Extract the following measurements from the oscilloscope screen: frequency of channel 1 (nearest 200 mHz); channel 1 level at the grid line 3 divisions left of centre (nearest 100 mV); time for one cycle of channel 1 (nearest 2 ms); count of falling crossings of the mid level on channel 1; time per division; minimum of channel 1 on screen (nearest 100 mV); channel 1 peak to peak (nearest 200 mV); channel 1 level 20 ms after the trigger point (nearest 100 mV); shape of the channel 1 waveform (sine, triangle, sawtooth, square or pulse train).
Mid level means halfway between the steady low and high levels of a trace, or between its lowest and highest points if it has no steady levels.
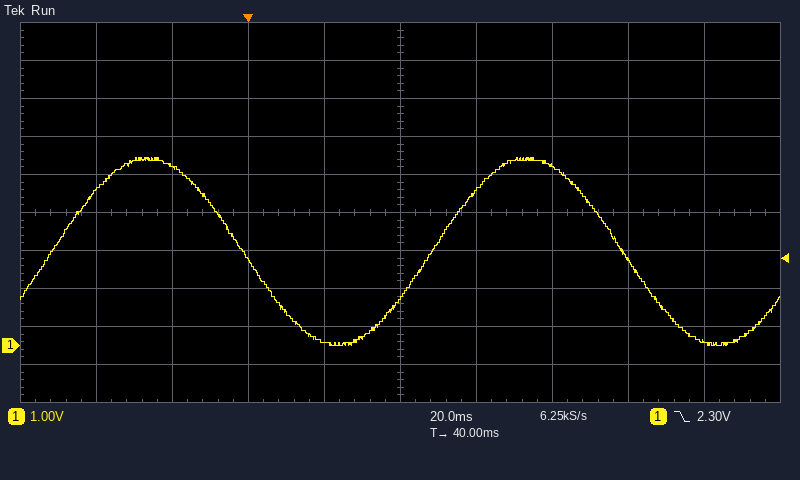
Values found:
10.0 Hz
4.7 V
100 ms
2
20 ms
0.0 V
5.0 V
100 mV
sine
